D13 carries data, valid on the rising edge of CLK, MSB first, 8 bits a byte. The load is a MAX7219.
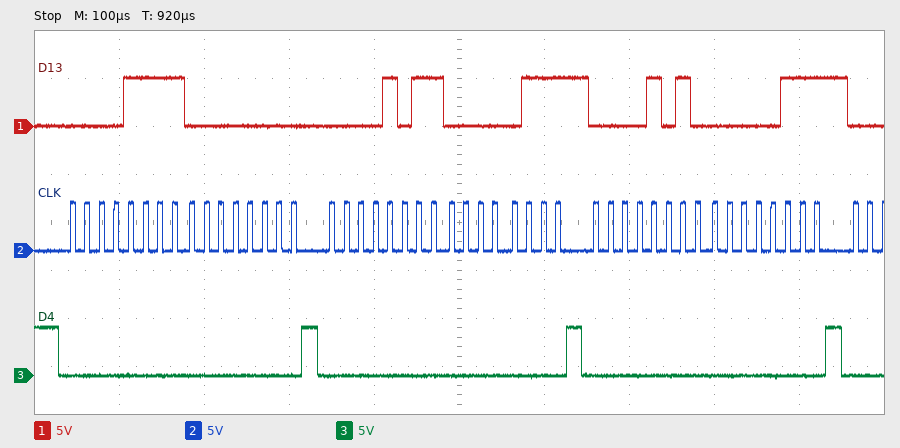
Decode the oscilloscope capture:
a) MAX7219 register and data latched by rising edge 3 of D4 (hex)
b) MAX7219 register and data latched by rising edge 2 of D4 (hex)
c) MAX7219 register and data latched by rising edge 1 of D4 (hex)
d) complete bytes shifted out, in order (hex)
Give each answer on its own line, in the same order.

register 0xA, data 0x07
register 0xB, data 0x07
register 0xF, data 0x00
0F 00 0B 07 0A 07
